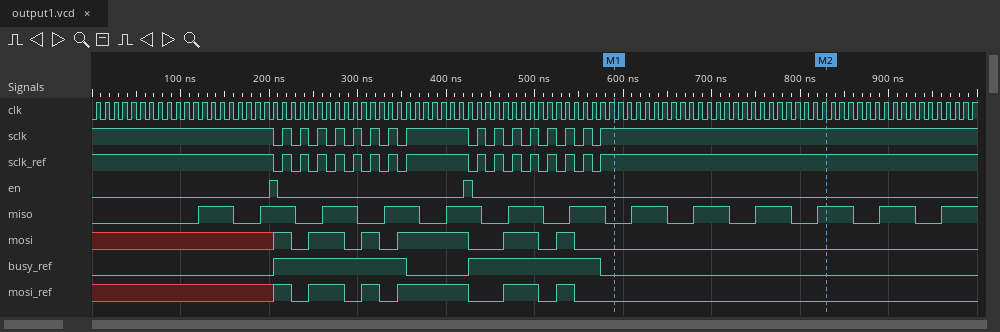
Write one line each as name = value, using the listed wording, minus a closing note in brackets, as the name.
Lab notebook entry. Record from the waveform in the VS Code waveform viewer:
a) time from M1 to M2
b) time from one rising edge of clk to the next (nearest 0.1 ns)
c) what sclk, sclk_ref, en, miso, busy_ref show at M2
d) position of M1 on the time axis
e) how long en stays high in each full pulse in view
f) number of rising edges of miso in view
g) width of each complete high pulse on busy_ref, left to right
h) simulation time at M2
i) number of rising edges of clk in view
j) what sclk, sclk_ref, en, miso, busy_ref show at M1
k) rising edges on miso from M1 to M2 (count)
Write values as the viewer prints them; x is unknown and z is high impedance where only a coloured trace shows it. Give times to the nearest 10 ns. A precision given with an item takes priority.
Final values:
time from M1 to M2 = 240 ns
time from one rising edge of clk to the next = 10 ns
what sclk, sclk_ref, en, miso, busy_ref show at M2 = sclk=1, sclk_ref=1, en=0, miso=1, busy_ref=0
position of M1 on the time axis = 590 ns
how long en stays high in each full pulse in view = 10 ns, 10 ns
number of rising edges of miso in view = 13
width of each complete high pulse on busy_ref, left to right = 150 ns, 150 ns
simulation time at M2 = 830 ns
number of rising edges of clk in view = 100
what sclk, sclk_ref, en, miso, busy_ref show at M1 = sclk=1, sclk_ref=1, en=0, miso=0, busy_ref=0
rising edges on miso from M1 to M2 = 4
